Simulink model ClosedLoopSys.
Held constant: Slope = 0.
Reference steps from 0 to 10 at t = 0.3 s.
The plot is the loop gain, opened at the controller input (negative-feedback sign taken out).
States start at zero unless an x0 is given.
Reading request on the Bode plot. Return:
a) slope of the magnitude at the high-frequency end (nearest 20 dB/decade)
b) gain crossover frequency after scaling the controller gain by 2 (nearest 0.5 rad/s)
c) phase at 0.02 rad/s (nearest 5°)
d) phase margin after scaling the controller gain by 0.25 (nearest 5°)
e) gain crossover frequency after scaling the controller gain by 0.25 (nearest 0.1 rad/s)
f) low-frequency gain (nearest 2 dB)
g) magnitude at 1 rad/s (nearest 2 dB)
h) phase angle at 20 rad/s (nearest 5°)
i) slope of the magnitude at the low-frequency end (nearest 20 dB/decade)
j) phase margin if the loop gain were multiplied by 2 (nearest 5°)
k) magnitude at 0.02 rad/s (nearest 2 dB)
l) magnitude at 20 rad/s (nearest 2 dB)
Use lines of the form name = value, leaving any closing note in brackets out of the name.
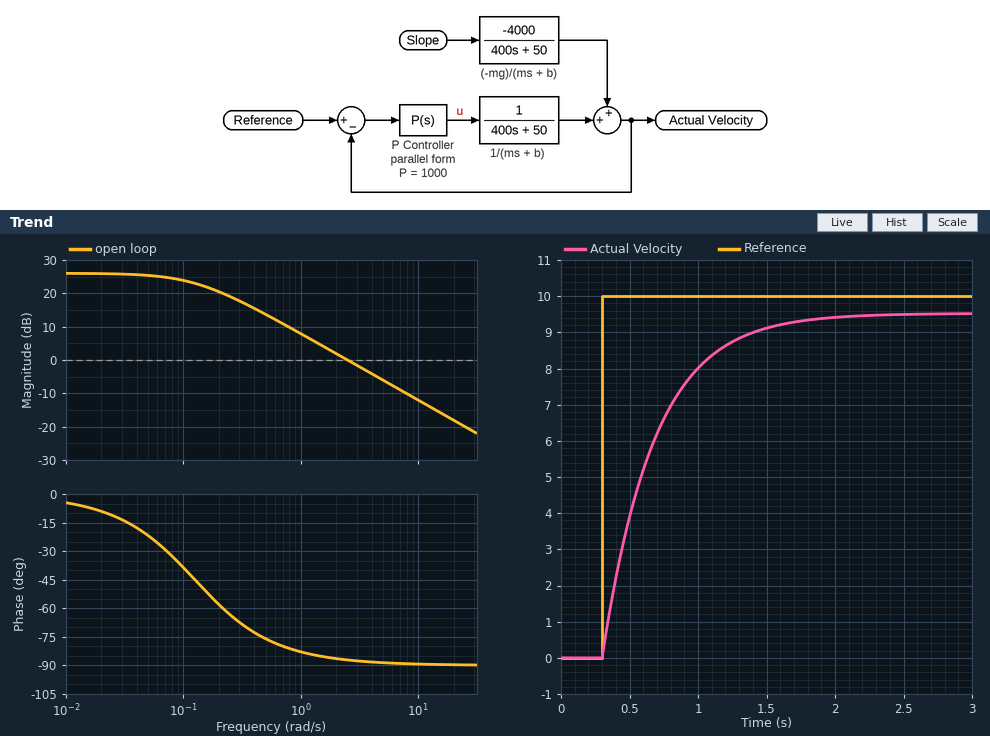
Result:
slope of the magnitude at the high-frequency end = -20 dB/decade
gain crossover frequency after scaling the controller gain by 2 = 5.0 rad/s
phase at 0.02 rad/s = -10°
phase margin after scaling the controller gain by 0.25 = 100°
gain crossover frequency after scaling the controller gain by 0.25 = 0.6 rad/s
low-frequency gain = 26 dB
magnitude at 1 rad/s = 8 dB
phase angle at 20 rad/s = -90°
slope of the magnitude at the low-frequency end = 0 dB/decade
phase margin if the loop gain were multiplied by 2 = 90°
magnitude at 0.02 rad/s = 26 dB
magnitude at 20 rad/s = -18 dB
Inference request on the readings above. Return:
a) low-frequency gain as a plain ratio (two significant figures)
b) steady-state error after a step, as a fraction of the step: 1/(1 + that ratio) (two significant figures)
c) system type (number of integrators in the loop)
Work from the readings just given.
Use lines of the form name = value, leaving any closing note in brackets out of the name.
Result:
low-frequency gain as a plain ratio = 20
steady-state error after a step, as a fraction of the step: 1/(1 + that ratio) = 0.048
system type = 0
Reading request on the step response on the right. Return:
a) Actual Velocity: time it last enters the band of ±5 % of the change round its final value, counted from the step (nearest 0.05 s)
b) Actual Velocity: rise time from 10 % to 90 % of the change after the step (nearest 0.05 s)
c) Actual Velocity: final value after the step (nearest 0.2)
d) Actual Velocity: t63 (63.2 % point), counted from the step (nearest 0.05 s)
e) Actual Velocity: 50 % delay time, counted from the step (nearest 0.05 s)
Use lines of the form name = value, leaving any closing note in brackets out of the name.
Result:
Actual Velocity: time it last enters the band of ±5 % of the change round its final value, counted from the step = 1.15 s
Actual Velocity: rise time from 10 % to 90 % of the change after the step = 0.85 s
Actual Velocity: final value after the step = 9.6
Actual Velocity: t63 (63.2 % point), counted from the step = 0.40 s
Actual Velocity: 50 % delay time, counted from the step = 0.25 s
